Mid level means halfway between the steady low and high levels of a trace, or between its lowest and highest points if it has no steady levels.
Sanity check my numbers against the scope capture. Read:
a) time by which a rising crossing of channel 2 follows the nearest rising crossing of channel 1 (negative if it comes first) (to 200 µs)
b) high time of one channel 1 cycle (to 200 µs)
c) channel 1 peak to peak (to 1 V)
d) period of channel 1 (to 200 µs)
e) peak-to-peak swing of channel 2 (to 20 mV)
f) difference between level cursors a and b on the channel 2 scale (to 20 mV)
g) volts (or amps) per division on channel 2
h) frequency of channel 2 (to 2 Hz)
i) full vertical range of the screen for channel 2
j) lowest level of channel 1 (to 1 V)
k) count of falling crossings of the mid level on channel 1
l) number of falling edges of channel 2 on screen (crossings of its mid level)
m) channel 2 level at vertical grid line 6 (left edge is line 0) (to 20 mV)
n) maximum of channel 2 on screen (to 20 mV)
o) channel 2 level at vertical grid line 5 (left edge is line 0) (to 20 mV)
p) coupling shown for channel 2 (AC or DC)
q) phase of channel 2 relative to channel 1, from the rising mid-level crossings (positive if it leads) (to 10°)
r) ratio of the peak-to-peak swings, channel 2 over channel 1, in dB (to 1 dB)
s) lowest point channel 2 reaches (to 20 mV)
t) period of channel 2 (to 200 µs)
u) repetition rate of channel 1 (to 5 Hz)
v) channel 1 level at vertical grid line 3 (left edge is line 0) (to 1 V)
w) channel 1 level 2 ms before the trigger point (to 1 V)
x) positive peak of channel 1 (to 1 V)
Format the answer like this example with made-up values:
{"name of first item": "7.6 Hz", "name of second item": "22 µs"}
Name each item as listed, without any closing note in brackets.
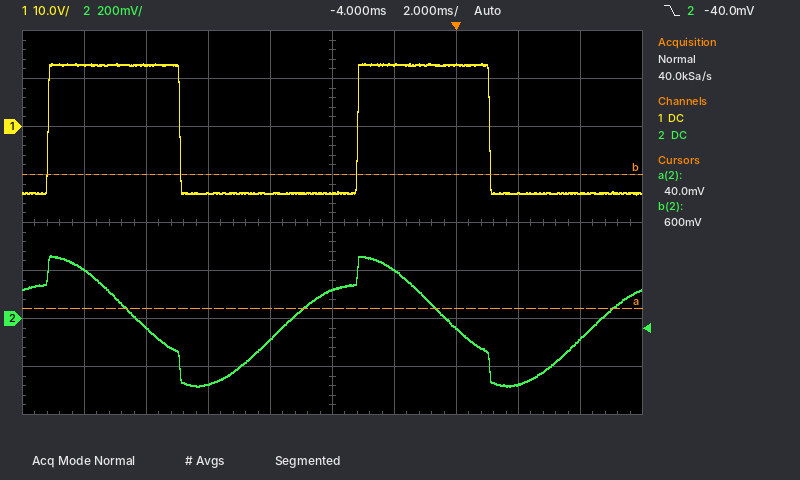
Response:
{"time by which a rising crossing of channel 2 follows the nearest rising crossing of channel 1 (negative if it comes first)": "-2.2 ms", "high time of one channel 1 cycle": "4.2 ms", "channel 1 peak to peak": "27 V", "period of channel 1": "10.0 ms", "peak-to-peak swing of channel 2": "540 mV", "difference between level cursors a and b on the channel 2 scale": "560 mV", "volts (or amps) per division on channel 2": "200 mV", "frequency of channel 2": "100 Hz", "full vertical range of the screen for channel 2": "1.6 V", "lowest level of channel 1": "-14 V", "count of falling crossings of the mid level on channel 1": "2", "number of falling edges of channel 2 on screen": "2", "channel 2 level at vertical grid line 6 (left edge is line 0)": "200 mV", "maximum of channel 2 on screen": "260 mV", "channel 2 level at vertical grid line 5 (left edge is line 0)": "120 mV", "coupling shown for channel 2": "DC", "phase of channel 2 relative to channel 1, from the rising mid-level crossings (positive if it leads)": "+80°", "ratio of the peak-to-peak swings, channel 2 over channel 1, in dB": "-34 dB", "lowest point channel 2 reaches": "-280 mV", "period of channel 2": "10.0 ms", "repetition rate of channel 1": "100 Hz", "channel 1 level at vertical grid line 3 (left edge is line 0)": "-14 V", "channel 1 level 2 ms before the trigger point": "13 V", "positive peak of channel 1": "13 V"}
